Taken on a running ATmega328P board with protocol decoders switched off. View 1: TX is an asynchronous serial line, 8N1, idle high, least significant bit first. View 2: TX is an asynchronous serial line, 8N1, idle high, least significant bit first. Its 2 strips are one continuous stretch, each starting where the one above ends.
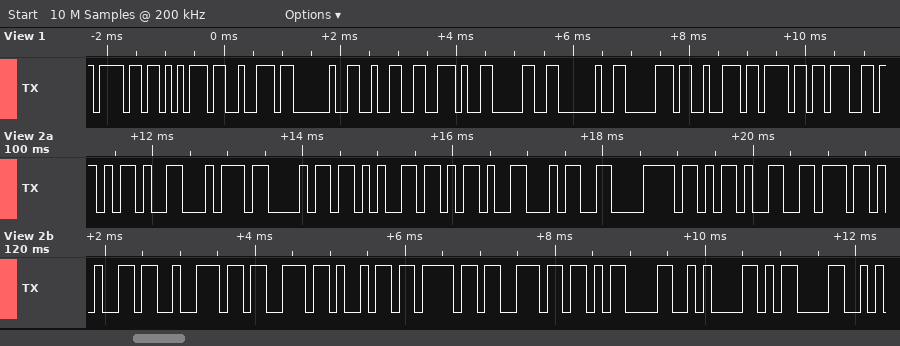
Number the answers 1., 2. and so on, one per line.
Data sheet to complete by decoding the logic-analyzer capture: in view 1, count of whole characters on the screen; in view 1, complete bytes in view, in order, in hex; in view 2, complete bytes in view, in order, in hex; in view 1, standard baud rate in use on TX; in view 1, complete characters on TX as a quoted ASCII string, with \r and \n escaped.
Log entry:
1. 12
2. 6F 75 72 20 32 2E 30 20 70 72 6F 67
3. 2D 74 68 65 2D 34 78 2D 76 65 72 73 69 6F 6E 0D 0A 0D
4. 9600 baud
5. "our 2.0 prog"
